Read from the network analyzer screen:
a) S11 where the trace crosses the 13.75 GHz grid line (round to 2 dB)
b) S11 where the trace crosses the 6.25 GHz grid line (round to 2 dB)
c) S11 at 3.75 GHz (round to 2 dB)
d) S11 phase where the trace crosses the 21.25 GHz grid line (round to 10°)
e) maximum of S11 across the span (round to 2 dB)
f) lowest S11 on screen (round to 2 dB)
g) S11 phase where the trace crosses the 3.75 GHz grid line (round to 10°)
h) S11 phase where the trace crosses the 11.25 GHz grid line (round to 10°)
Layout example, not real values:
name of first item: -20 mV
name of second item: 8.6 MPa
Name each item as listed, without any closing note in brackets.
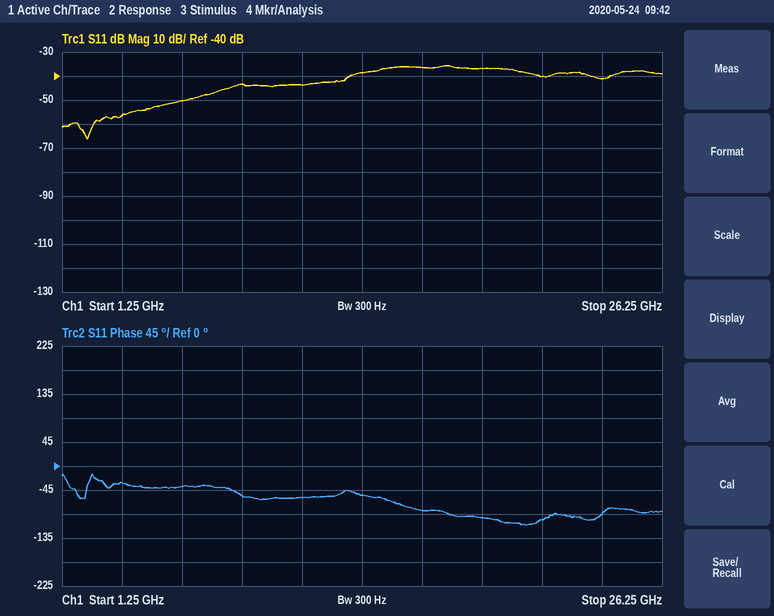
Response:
S11 where the trace crosses the 13.75 GHz grid line: -38 dB
S11 where the trace crosses the 6.25 GHz grid line: -50 dB
S11 at 3.75 GHz: -56 dB
S11 phase where the trace crosses the 21.25 GHz grid line: -100°
maximum of S11 across the span: -36 dB
lowest S11 on screen: -66 dB
S11 phase where the trace crosses the 3.75 GHz grid line: -30°
S11 phase where the trace crosses the 11.25 GHz grid line: -60°
